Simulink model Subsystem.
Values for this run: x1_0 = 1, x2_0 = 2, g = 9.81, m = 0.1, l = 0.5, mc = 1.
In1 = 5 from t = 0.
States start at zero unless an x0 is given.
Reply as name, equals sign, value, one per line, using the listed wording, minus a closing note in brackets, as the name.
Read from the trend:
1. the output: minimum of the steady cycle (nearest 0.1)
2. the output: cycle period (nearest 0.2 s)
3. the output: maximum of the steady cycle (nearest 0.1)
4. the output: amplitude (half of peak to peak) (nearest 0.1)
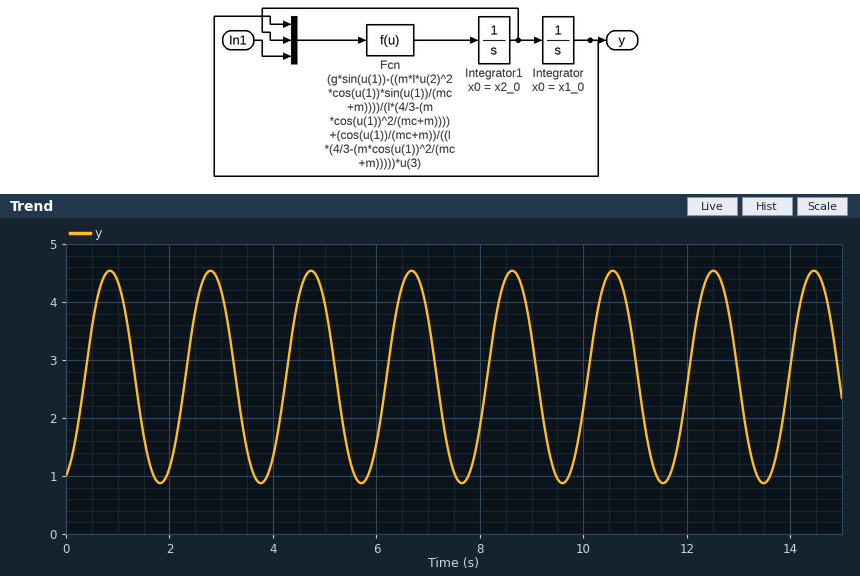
the output: minimum of the steady cycle = 0.9
the output: cycle period = 2.0 s
the output: maximum of the steady cycle = 4.5
the output: amplitude (half of peak to peak) = 1.8
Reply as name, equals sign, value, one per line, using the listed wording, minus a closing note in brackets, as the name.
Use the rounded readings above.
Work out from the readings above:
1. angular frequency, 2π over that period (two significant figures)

angular frequency, 2π over that period = 3.1 rad/s
